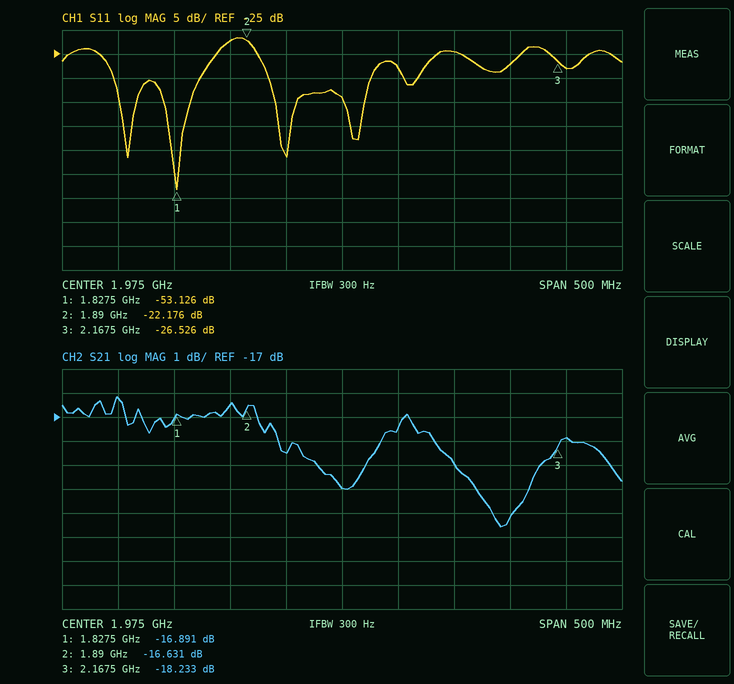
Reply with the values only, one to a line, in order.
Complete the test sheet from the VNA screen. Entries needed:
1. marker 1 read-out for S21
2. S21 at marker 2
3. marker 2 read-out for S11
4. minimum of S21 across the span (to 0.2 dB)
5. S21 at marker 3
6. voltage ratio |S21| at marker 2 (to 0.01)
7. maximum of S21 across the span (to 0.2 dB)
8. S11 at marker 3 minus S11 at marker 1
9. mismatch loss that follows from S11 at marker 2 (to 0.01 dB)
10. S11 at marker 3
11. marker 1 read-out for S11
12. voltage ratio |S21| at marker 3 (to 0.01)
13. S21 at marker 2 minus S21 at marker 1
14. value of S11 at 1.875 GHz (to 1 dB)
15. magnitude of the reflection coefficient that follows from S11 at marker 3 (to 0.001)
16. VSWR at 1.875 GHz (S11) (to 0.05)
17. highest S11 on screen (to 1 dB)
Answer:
-16.891 dB
-16.631 dB
-22.176 dB
-21.6 dB
-18.233 dB
0.15
-16.2 dB
26.600 dB
0.03 dB
-26.526 dB
-53.126 dB
0.12
0.260 dB
-22 dB
0.047
1.15
-22 dB
